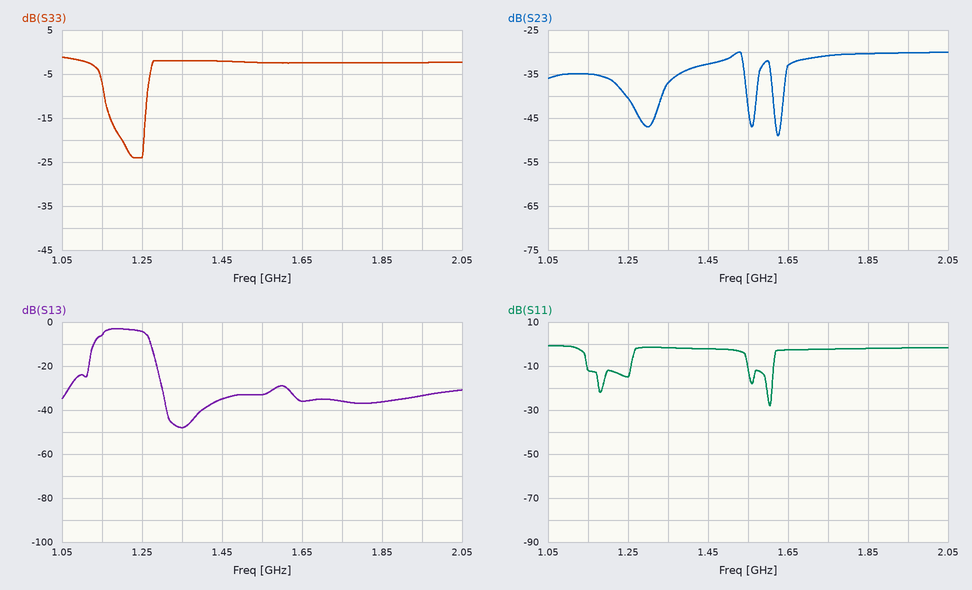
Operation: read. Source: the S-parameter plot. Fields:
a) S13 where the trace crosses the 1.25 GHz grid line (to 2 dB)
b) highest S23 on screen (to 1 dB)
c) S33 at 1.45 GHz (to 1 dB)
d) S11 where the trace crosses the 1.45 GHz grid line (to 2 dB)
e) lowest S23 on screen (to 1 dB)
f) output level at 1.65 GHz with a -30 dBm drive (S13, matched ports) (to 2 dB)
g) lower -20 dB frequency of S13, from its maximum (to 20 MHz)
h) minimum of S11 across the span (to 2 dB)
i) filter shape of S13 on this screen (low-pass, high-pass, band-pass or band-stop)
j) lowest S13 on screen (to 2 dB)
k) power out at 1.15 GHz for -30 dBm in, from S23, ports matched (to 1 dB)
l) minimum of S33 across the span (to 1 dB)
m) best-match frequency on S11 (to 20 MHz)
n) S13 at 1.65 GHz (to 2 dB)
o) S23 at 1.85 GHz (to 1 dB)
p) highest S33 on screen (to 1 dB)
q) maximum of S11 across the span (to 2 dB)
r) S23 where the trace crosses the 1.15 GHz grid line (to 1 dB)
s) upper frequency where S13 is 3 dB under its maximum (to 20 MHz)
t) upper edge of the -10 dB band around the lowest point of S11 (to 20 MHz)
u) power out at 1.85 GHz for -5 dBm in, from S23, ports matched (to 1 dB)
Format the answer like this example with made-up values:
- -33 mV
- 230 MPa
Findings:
- -4 dB
- -30 dB
- -2 dB
- -2 dB
- -49 dB
- -66 dBm
- 1.12 GHz
- -28 dB
- band-pass
- -48 dB
- -65 dBm
- -24 dB
- 1.60 GHz
- -36 dB
- -30 dB
- -1 dB
- 0 dB
- -35 dB
- 1.26 GHz
- 1.62 GHz
- -35 dBm
